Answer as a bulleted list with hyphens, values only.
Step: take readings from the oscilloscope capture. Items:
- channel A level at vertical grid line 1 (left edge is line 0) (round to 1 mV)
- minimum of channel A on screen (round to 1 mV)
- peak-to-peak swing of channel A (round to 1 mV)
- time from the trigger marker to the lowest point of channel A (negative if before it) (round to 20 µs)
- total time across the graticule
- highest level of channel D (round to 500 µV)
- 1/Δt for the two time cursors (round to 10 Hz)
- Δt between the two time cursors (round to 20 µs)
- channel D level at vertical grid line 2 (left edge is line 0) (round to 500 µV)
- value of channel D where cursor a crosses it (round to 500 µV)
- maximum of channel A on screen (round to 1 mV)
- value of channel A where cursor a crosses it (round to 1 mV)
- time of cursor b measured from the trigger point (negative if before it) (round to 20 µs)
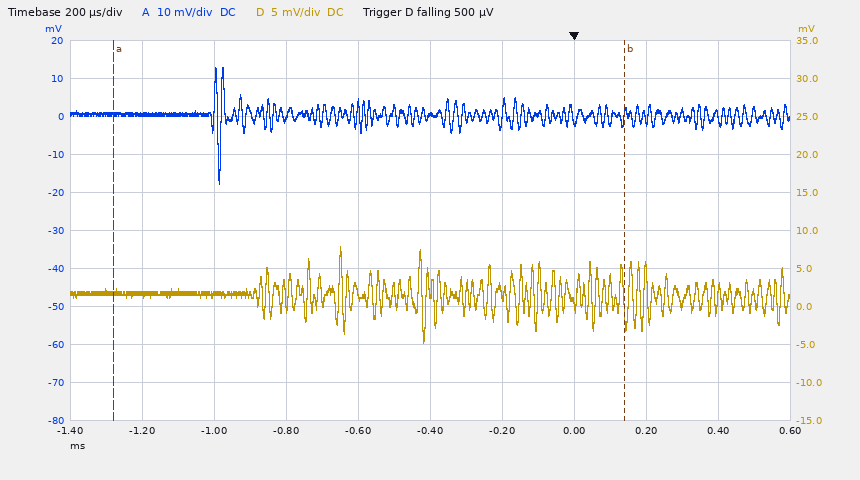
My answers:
- 1 mV
- -18 mV
- 31 mV
- -980 µs
- 2 ms
- 8.0 mV
- 700 Hz
- 1.42 ms
- 1.5 mV
- 2.0 mV
- 13 mV
- 1 mV
- +140 µs
